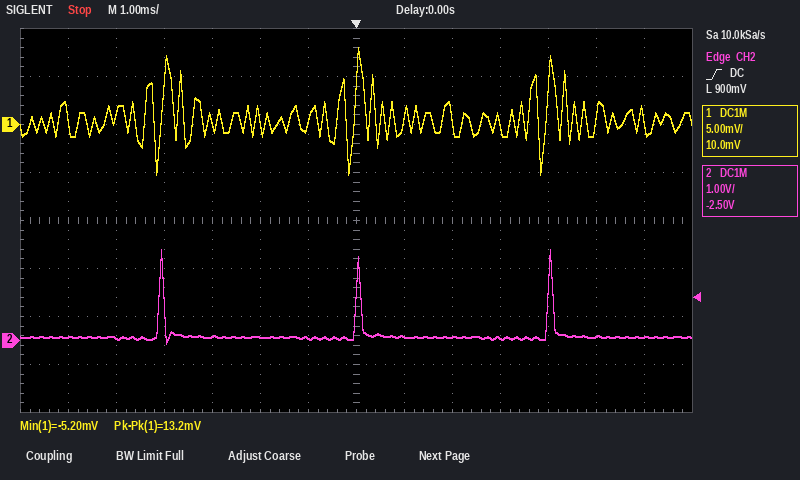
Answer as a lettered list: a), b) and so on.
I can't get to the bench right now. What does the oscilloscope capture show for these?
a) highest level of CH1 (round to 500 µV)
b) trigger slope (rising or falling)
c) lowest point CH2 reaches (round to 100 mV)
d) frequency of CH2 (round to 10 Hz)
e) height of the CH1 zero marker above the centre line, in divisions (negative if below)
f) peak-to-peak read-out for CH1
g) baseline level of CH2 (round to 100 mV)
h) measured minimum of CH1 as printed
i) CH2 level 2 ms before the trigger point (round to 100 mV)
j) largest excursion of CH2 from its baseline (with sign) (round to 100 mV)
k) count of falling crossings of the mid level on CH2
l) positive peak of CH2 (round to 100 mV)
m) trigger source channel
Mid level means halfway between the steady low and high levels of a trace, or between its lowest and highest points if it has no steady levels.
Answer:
a) 8.0 mV
b) rising
c) -100 mV
d) 250 Hz
e) +2.0 div
f) 13.2 mV
g) 100 mV
h) -5.20 mV
i) 100 mV
j) +1.8 V
k) 3
l) 1.9 V
m) CH2
